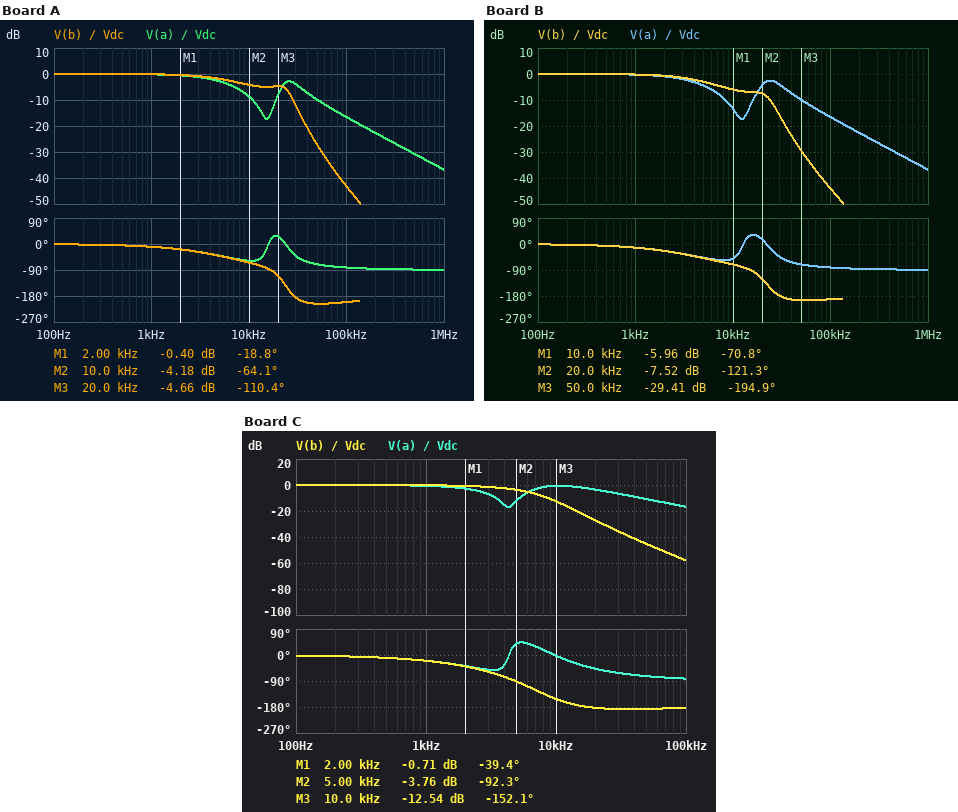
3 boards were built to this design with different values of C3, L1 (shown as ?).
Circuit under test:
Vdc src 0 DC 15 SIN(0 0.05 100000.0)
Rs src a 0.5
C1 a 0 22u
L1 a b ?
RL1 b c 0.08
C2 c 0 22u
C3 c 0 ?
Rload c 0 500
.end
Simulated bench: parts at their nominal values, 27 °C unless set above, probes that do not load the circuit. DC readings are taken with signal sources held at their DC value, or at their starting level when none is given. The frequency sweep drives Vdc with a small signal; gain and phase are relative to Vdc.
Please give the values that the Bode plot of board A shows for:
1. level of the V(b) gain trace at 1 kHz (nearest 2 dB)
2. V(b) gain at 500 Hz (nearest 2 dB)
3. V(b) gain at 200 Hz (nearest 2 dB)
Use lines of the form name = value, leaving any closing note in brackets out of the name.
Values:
level of the V(b) gain trace at 1 kHz = 0 dB
V(b) gain at 500 Hz = 0 dB
V(b) gain at 200 Hz = 0 dB
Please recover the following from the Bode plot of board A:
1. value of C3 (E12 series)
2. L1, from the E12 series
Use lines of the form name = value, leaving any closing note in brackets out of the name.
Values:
value of C3 = 10 µF
L1, from the E12 series = 3.3 µH
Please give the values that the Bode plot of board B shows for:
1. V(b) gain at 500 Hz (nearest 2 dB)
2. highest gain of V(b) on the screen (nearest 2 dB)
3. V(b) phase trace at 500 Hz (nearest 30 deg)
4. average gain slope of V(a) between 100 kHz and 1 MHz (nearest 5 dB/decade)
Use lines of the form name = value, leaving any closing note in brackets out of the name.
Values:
V(b) gain at 500 Hz = 0 dB
highest gain of V(b) on the screen = 0 dB
V(b) phase trace at 500 Hz = 0 deg
average gain slope of V(a) between 100 kHz and 1 MHz = -20 dB/decade
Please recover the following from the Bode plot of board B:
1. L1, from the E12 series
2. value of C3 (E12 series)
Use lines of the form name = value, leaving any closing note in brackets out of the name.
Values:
L1, from the E12 series = 3.3 µH
value of C3 = 27 µF
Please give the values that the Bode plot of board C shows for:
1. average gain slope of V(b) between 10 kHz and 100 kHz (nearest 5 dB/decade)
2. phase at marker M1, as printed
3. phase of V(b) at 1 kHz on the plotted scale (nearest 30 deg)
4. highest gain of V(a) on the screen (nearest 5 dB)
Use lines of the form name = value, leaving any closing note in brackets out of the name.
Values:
average gain slope of V(b) between 10 kHz and 100 kHz = -45 dB/decade
phase at marker M1, as printed = -39.4 deg
phase of V(b) at 1 kHz on the plotted scale = -30 deg
highest gain of V(a) on the screen = 0 dB
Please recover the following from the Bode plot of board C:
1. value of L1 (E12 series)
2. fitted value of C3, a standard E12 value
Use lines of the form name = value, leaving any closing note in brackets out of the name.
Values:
value of L1 = 15 µH
fitted value of C3, a standard E12 value = 68 µF
